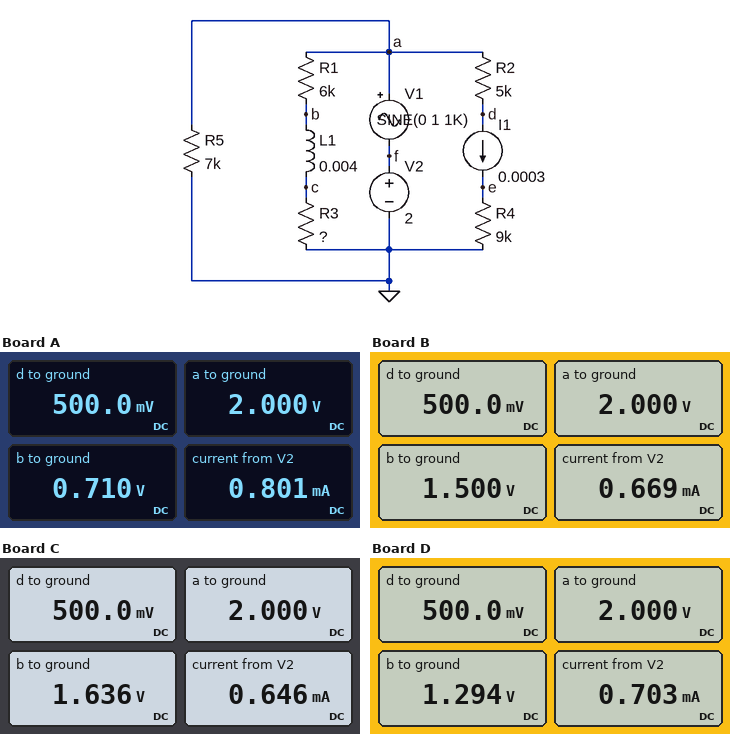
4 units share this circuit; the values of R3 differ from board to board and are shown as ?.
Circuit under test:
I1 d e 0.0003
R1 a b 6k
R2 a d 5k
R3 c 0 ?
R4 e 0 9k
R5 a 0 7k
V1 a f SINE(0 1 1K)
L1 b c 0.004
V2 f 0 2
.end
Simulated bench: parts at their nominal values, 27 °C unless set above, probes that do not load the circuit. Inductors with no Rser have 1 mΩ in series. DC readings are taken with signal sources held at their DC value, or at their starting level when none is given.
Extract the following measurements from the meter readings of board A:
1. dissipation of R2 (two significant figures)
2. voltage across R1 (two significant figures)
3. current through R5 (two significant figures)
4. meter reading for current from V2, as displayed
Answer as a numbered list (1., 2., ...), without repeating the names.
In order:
1. 450 µW
2. 1.3 V
3. 290 µA
4. 0.801 mA
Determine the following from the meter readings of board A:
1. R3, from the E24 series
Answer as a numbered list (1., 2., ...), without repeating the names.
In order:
1. 3.3 kΩ
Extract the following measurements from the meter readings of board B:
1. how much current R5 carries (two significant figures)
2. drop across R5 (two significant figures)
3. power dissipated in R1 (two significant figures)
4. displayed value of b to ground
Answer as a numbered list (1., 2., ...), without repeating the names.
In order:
1. 290 µA
2. 2.0 V
3. 42 µW
4. 1.500 V
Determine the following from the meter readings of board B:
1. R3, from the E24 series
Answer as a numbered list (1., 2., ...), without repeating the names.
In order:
1. 18 kΩ
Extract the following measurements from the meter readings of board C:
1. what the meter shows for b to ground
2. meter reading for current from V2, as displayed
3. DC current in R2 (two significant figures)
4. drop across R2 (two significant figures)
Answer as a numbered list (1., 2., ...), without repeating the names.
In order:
1. 1.636 V
2. 0.646 mA
3. 300 µA
4. 1.5 V
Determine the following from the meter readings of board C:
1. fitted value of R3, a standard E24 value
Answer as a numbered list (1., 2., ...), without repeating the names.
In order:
1. 27 kΩ
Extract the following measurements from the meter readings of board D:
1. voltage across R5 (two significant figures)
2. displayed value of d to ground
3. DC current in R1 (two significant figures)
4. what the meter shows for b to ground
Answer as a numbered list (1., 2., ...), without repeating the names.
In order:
1. 2.0 V
2. 500.0 mV
3. 120 µA
4. 1.294 V
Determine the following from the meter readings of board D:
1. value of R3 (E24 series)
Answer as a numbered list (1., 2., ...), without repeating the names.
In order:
1. 11 kΩ
